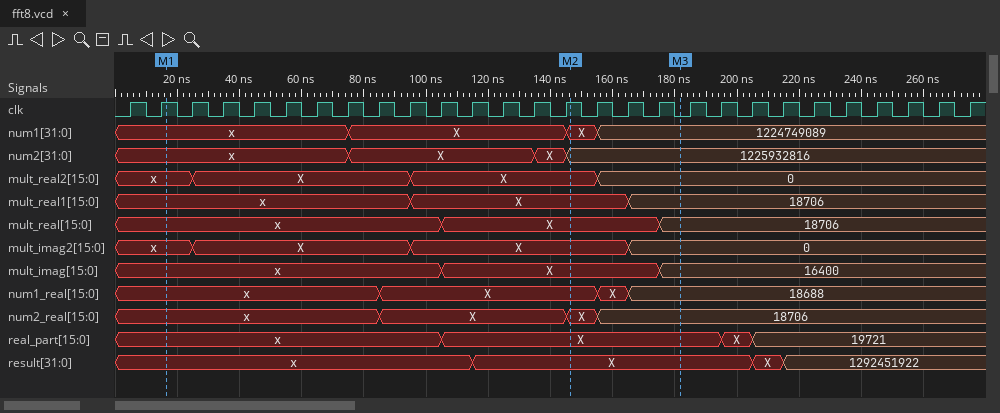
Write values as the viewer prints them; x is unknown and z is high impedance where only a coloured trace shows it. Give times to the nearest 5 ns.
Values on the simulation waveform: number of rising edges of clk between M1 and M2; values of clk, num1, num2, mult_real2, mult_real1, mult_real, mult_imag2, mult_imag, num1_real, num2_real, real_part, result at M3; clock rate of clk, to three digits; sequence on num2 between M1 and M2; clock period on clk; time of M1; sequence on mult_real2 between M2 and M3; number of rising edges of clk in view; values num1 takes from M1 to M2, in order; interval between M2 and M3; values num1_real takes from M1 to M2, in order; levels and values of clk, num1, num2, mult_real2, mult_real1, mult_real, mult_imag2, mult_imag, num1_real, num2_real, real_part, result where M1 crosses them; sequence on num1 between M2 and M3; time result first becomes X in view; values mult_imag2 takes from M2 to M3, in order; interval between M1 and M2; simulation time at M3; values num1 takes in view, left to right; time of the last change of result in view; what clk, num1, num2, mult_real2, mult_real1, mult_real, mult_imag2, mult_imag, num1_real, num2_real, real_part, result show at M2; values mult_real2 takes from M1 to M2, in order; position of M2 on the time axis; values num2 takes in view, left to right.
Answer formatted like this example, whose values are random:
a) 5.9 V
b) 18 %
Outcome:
a) 13
b) clk=0, num1=1224749089, num2=1225932816, mult_real2=0, mult_real1=18706, mult_real=18706, mult_imag2=0, mult_imag=16400, num1_real=18688, num2_real=18706, real_part=X, result=X
c) 100 MHz
d) x, X, X, 1225932816
e) 10 ns
f) 15 ns
g) X, 0
h) 28
i) x, X, X
j) 35 ns
k) x, X
l) clk=1, num1=x, num2=x, mult_real2=x, mult_real1=x, mult_real=x, mult_imag2=x, mult_imag=x, num1_real=x, num2_real=x, real_part=x, result=x
m) X, 1224749089
n) 115 ns
o) X, 0
p) 130 ns
q) 180 ns
r) x, X, X, 1224749089
s) 215 ns
t) clk=1, num1=X, num2=1225932816, mult_real2=X, mult_real1=X, mult_real=X, mult_imag2=X, mult_imag=X, num1_real=X, num2_real=X, real_part=X, result=X
u) x, X, X
v) 145 ns
w) x, X, X, 1225932816
